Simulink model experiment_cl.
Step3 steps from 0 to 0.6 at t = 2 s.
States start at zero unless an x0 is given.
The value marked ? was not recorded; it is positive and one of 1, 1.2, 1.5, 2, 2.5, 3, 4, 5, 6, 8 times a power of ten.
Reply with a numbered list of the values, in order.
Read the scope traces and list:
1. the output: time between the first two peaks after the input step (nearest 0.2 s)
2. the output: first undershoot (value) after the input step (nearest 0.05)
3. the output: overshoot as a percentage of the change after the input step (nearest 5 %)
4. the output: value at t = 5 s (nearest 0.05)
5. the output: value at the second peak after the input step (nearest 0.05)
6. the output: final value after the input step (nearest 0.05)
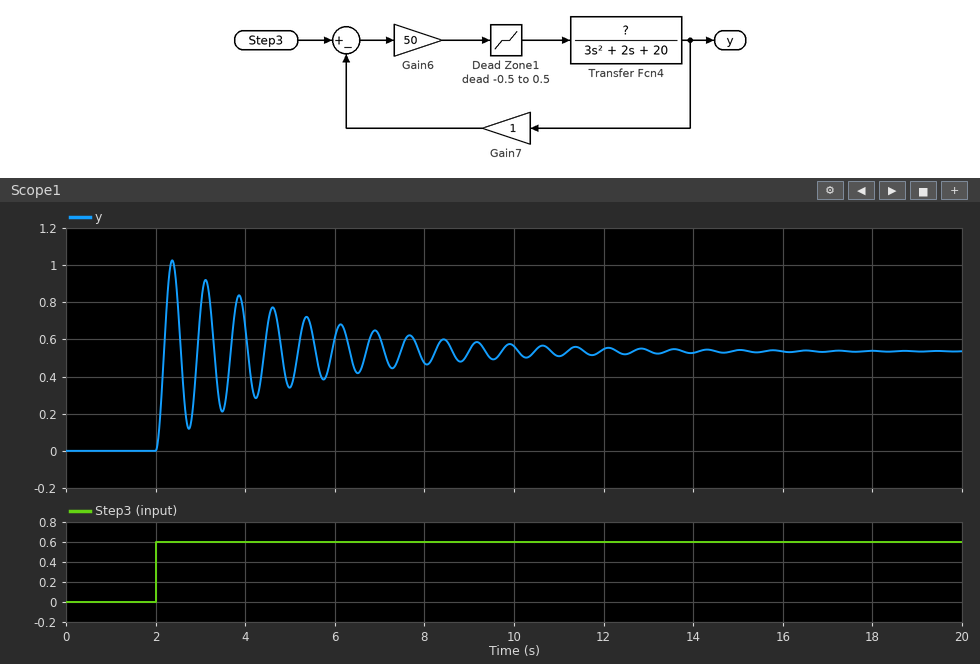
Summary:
1. 0.8 s
2. 0.10
3. 90 %
4. 0.35
5. 0.90
6. 0.55
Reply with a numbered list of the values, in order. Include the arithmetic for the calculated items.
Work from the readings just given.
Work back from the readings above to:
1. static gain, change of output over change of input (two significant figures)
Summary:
1. (0.55 - 0) / (0.6 - 0) = 0.92
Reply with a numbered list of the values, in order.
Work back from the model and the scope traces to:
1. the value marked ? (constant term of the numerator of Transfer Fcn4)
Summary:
1. 4
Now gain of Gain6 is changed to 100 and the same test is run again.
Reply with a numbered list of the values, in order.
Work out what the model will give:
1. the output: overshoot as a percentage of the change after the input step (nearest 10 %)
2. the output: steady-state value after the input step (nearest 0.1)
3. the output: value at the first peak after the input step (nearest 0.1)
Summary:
1. 90 %
2. 0.6
3. 1.1
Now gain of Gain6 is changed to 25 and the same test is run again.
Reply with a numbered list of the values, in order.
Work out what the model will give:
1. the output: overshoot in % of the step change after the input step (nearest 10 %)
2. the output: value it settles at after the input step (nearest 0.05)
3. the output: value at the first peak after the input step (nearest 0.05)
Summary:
1. 90 %
2. 0.50
3. 0.90
